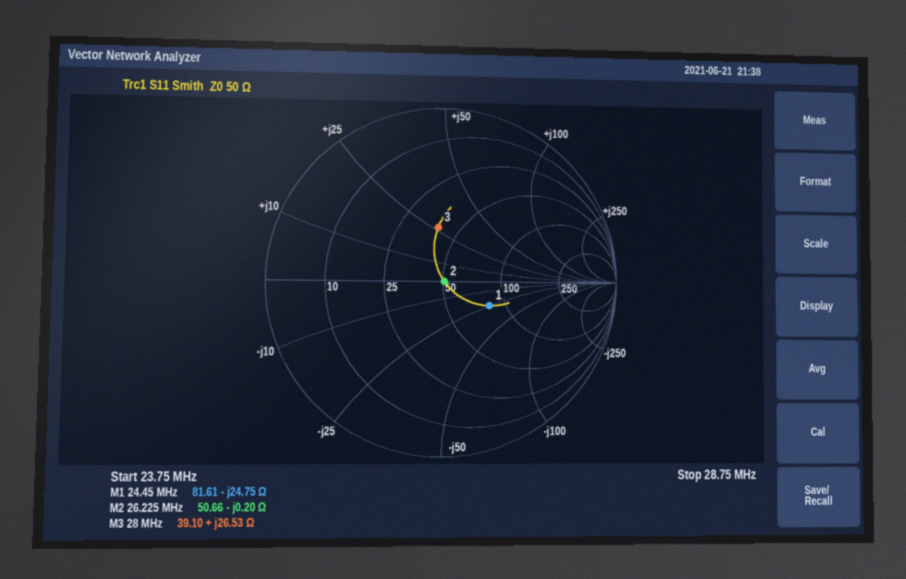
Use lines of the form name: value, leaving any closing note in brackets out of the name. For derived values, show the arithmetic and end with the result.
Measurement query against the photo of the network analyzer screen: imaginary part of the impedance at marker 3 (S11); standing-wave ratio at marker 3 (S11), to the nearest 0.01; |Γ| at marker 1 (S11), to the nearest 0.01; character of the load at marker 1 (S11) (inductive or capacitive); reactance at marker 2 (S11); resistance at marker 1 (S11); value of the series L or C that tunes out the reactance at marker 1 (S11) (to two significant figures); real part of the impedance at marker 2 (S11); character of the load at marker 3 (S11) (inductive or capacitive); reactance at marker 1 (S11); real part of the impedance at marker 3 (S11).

imaginary part of the impedance at marker 3: +26.53 Ω
standing-wave ratio at marker 3 (S11), to the nearest 0.01: 1.89
|Γ| at marker 1 (S11), to the nearest 0.01: 0.30
character of the load at marker 1 (S11): capacitive
reactance at marker 2: -0.20 Ω
resistance at marker 1: 81.61 Ω
value of the series L or C that tunes out the reactance at marker 1 (S11): L = 24.75 Ω/(2π × 24.45 MHz) ≈ 161 nH, so 160 nH to two significant figures
real part of the impedance at marker 2: 50.66 Ω
character of the load at marker 3 (S11): inductive
reactance at marker 1: -24.75 Ω
real part of the impedance at marker 3: 39.10 Ω
